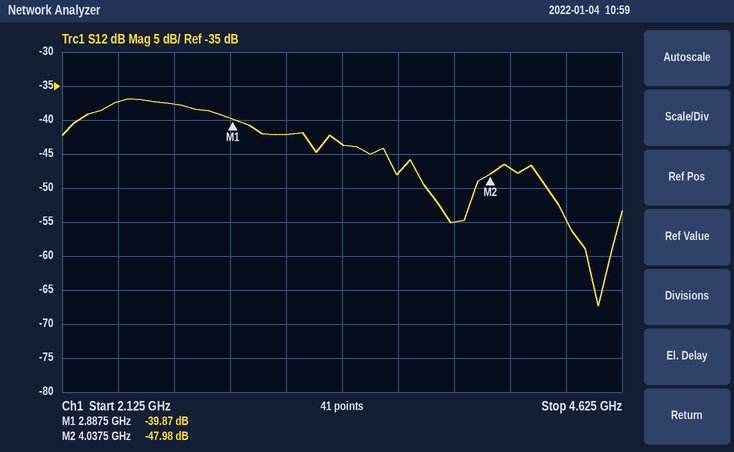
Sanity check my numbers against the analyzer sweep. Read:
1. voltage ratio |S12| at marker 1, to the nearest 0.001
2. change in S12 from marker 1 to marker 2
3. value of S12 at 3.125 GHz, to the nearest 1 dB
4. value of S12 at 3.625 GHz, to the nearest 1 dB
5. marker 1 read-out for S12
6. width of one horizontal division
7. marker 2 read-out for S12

0.010
-8.11 dB
-42 dB
-48 dB
-39.87 dB
250 MHz
-47.98 dB
